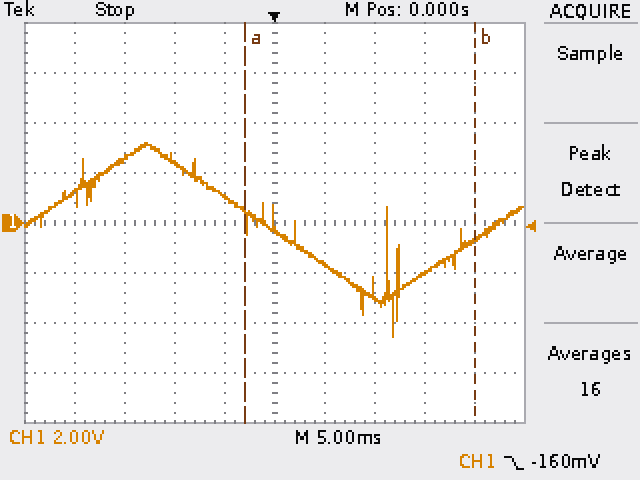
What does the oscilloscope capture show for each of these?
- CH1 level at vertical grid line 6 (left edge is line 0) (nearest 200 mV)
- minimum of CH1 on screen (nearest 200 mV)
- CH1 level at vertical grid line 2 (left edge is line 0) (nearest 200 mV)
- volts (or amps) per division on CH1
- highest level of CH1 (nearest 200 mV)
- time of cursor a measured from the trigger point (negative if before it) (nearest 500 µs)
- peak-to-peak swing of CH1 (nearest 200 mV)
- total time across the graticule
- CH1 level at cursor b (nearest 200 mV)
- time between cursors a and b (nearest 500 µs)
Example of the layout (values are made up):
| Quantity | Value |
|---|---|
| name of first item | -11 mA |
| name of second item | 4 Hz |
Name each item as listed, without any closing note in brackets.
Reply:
| Quantity | Value |
|---|---|
| CH1 level at vertical grid line 6 (left edge is line 0) | -1.6 V |
| minimum of CH1 on screen | -4.6 V |
| CH1 level at vertical grid line 2 (left edge is line 0) | 2.6 V |
| volts (or amps) per division on CH1 | 2 V |
| highest level of CH1 | 3.2 V |
| time of cursor a measured from the trigger point (negative if before it) | -3.0 ms |
| peak-to-peak swing of CH1 | 7.8 V |
| total time across the graticule | 50 ms |
| CH1 level at cursor b | -600 mV |
| time between cursors a and b | 23.0 ms |
